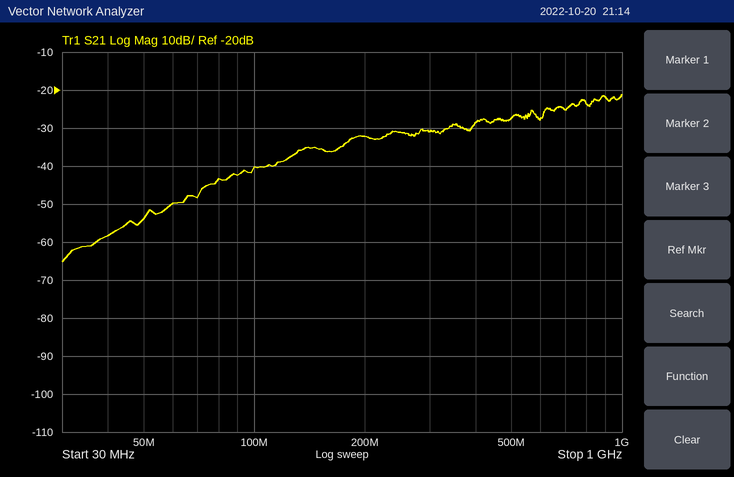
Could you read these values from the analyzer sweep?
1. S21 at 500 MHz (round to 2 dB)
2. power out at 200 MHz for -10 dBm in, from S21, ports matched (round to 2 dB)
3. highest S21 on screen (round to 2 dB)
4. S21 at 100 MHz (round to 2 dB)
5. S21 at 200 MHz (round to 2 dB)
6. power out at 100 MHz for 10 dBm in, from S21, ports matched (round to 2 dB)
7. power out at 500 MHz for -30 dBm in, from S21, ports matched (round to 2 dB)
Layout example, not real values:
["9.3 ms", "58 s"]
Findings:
["-28 dB", "-42 dBm", "-22 dB", "-40 dB", "-32 dB", "-30 dBm", "-58 dBm"]
